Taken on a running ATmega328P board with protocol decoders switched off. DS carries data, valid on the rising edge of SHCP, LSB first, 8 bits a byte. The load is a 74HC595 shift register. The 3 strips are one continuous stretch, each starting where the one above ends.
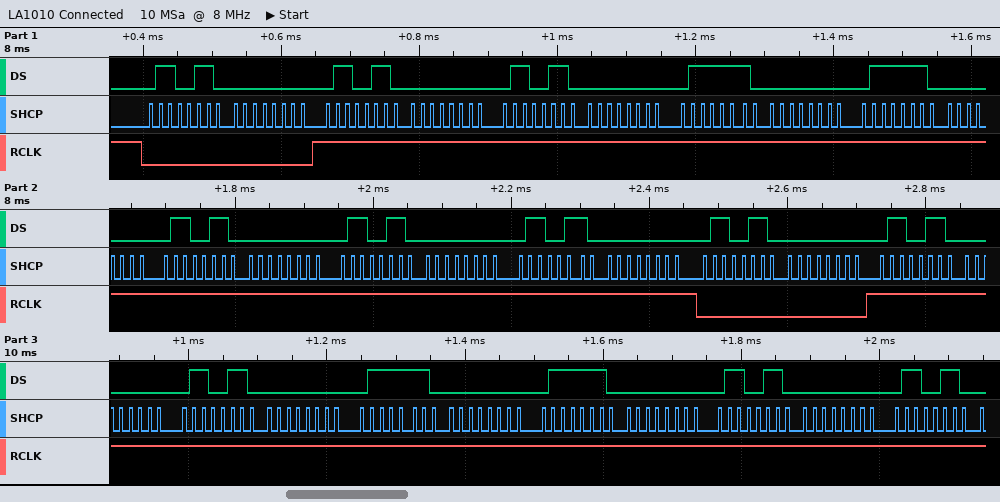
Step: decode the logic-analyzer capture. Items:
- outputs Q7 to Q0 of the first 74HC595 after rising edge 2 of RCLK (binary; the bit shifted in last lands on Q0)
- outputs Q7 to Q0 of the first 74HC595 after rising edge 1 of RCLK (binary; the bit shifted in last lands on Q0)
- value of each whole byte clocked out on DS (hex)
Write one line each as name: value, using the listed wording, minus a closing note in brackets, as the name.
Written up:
outputs Q7 to Q0 of the first 74HC595 after rising edge 2 of RCLK: 00000000
outputs Q7 to Q0 of the first 74HC595 after rising edge 1 of RCLK: 00000000
value of each whole byte clocked out on DS: 66 00 66 00 66 00 7E 00 7E 00 66 00 66 00 66 00 66 00 66 00 66 00 7E 00 7E 00 66 00 66
